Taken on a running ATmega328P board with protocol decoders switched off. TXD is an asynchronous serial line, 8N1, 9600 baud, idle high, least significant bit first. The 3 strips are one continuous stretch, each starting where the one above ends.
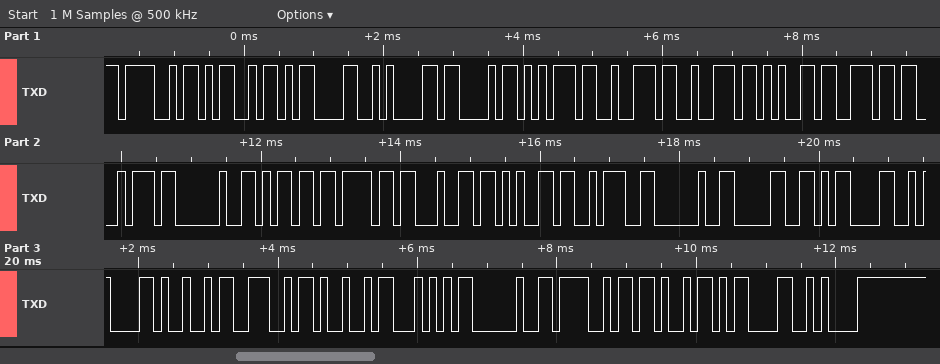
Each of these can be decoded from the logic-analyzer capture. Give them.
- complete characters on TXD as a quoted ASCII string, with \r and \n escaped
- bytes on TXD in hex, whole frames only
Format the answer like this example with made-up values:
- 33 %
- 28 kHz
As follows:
- "OM\r\nCurrent mode: 0\r\nINIT OK\r\n"
- 4F 4D 0D 0A 43 75 72 72 65 6E 74 20 6D 6F 64 65 3A 20 30 0D 0A 49 4E 49 54 20 4F 4B 0D 0A
